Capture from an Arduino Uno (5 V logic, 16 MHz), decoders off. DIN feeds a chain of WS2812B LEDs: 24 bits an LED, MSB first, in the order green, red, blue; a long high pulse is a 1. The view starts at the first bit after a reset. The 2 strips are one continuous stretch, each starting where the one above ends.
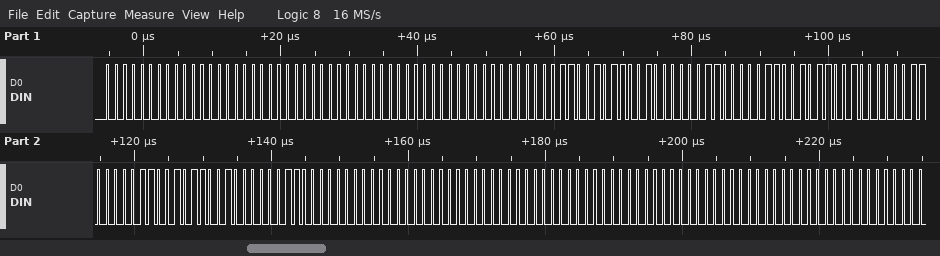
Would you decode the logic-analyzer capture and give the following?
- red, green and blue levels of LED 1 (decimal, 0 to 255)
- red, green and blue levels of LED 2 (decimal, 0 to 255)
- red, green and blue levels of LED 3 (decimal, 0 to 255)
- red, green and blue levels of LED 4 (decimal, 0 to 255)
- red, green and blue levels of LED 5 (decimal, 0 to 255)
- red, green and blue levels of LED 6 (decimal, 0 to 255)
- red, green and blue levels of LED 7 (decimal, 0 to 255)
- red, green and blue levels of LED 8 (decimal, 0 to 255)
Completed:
0, 0, 0
0, 0, 0
89, 6, 3
89, 6, 3
89, 6, 3
0, 0, 0
0, 0, 0
0, 0, 0
